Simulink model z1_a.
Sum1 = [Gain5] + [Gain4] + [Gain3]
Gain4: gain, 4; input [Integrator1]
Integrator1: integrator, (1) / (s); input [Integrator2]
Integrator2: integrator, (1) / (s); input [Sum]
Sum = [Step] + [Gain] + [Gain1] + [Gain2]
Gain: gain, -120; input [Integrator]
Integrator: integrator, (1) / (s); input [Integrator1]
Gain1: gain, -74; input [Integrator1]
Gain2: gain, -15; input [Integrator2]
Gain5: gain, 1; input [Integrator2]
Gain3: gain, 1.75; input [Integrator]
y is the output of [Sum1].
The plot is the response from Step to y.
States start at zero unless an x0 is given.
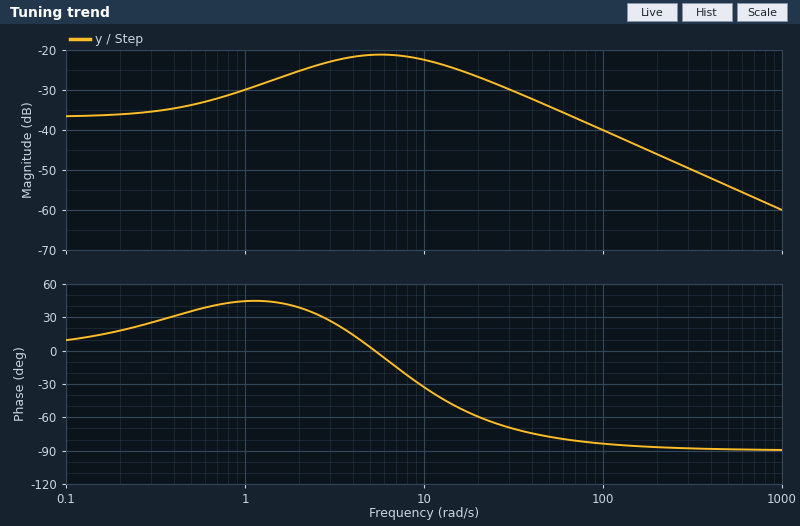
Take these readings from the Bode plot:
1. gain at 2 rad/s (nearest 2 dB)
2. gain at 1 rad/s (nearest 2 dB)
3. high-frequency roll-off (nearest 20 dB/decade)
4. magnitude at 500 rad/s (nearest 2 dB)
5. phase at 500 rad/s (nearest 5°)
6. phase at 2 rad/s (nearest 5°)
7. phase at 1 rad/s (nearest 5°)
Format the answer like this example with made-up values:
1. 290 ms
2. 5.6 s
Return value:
1. -26 dB
2. -30 dB
3. -20 dB/decade
4. -54 dB
5. -90°
6. 40°
7. 45°
